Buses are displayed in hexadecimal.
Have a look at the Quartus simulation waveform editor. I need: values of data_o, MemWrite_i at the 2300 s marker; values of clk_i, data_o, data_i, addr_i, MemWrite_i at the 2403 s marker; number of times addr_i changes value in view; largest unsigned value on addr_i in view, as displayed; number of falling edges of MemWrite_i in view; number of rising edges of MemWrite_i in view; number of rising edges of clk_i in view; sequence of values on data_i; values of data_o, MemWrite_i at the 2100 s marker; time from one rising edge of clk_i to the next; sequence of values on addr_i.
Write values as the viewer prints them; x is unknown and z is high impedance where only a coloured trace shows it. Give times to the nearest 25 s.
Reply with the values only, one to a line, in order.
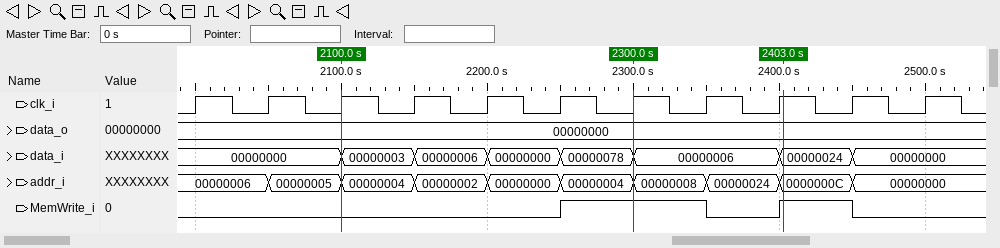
data_o=00000000, MemWrite_i=1
clk_i=1, data_o=00000000, data_i=00000024, addr_i=0000000C, MemWrite_i=1
9
00000024
2
2
11
00000000, 00000003, 00000006, 00000000, 00000078, 00000006, 00000024, 00000000
data_o=00000000, MemWrite_i=0
50 s
00000006, 00000005, 00000004, 00000002, 00000000, 00000004, 00000008, 00000024, 0000000C, 00000000
